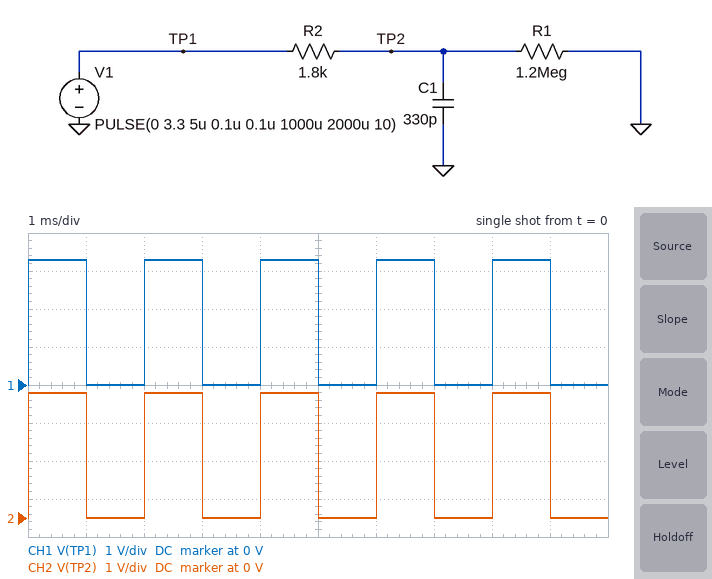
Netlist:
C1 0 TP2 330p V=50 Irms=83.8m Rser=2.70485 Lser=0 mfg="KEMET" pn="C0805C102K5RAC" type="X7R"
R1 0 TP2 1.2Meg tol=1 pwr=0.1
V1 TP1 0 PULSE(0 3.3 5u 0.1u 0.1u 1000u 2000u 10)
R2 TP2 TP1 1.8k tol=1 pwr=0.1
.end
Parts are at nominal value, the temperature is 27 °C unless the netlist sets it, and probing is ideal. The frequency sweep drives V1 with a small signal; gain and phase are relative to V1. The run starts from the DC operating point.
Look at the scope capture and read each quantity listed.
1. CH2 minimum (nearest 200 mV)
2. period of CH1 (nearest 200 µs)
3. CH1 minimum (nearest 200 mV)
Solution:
0 V
2.0 ms
0 V
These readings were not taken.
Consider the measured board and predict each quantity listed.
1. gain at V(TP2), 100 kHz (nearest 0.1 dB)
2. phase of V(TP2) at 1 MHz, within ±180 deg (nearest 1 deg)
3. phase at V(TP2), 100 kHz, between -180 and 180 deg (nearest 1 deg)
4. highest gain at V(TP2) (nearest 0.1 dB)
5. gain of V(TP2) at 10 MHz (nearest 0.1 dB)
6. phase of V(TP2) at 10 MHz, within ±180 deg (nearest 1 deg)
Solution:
-0.6 dB
-75 deg
-20 deg
0 dB
-31.4 dB
-85 deg
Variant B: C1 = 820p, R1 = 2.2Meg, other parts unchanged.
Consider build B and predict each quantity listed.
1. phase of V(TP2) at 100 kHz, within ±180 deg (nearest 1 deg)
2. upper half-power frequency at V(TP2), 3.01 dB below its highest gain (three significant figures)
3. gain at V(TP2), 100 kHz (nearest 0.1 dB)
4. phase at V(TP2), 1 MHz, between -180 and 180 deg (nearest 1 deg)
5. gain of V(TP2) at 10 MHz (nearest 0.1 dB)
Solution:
-43 deg
108 kHz
-2.7 dB
-83 deg
-39.3 dB
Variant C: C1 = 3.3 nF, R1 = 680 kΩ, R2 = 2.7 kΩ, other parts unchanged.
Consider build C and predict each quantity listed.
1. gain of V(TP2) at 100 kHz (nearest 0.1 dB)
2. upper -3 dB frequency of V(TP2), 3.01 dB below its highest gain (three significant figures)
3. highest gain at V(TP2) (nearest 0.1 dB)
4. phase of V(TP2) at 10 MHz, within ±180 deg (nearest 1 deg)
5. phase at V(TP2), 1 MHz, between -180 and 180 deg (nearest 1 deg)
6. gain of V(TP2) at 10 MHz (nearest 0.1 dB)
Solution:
-15.1 dB
17.9 kHz
0 dB
-61 deg
-86 deg
-53.8 dB
